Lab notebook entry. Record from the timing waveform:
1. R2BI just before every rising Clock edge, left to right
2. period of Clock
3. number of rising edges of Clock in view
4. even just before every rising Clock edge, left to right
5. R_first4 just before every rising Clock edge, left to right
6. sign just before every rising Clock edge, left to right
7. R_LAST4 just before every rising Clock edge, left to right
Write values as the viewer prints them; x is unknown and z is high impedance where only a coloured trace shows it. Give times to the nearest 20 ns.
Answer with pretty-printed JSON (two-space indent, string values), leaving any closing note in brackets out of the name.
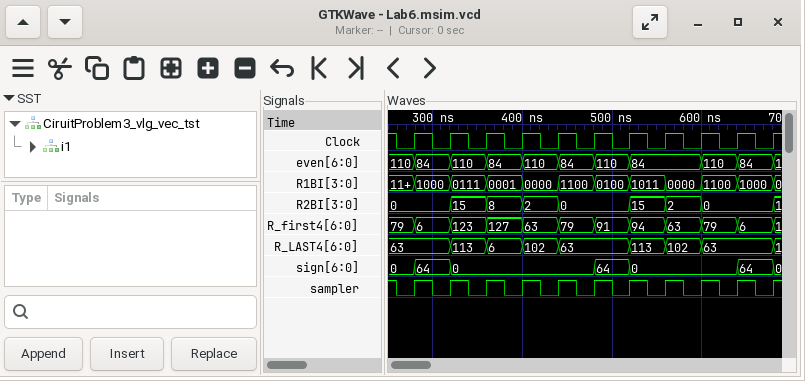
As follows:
{
  "R2BI just before every rising Clock edge, left to right": "0, 0, 15, 8, 2, 0, 0, 15, 2, 0, 0",
  "period of Clock": "40 ns",
  "number of rising edges of Clock in view": "11",
  "even just before every rising Clock edge, left to right": "110, 84, 110, 84, 110, 84, 110, 84, 84, 110, 84",
  "R_first4 just before every rising Clock edge, left to right": "79, 6, 123, 127, 63, 79, 91, 94, 63, 79, 6",
  "sign just before every rising Clock edge, left to right": "0, 64, 0, 0, 0, 0, 64, 0, 0, 0, 64",
  "R_LAST4 just before every rising Clock edge, left to right": "63, 63, 113, 6, 102, 63, 63, 113, 102, 63, 63"
}
